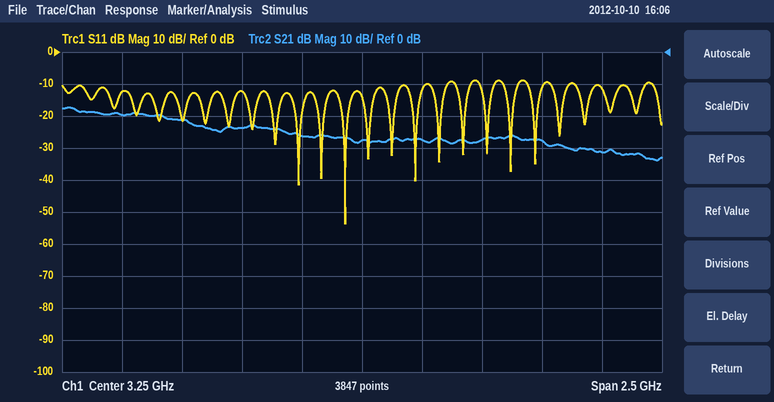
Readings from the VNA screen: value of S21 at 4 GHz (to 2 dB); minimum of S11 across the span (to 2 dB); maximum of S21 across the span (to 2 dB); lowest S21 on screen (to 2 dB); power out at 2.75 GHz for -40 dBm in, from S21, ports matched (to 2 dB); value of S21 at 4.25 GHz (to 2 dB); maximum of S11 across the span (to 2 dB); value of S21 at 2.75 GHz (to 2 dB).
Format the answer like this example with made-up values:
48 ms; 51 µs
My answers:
-28 dB; -54 dB; -18 dB; -34 dB; -64 dBm; -32 dB; -8 dB; -24 dB
